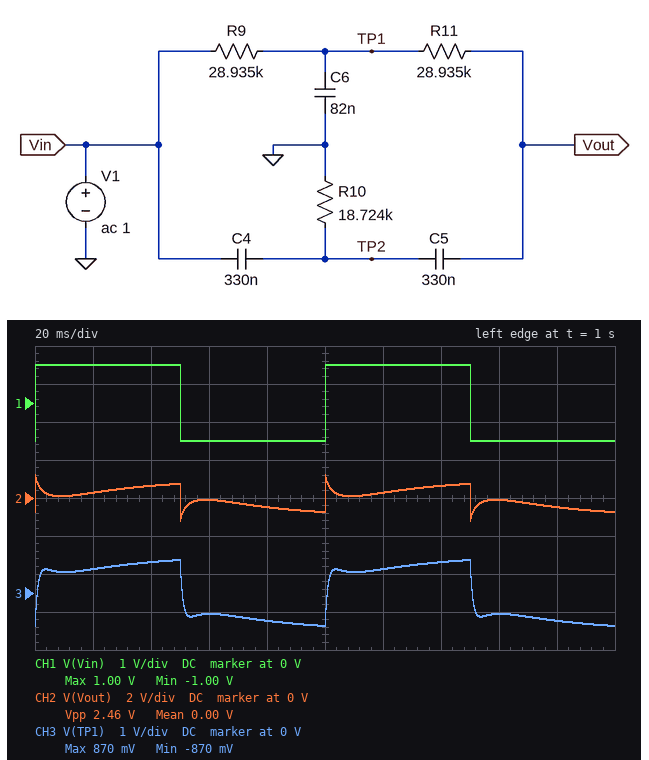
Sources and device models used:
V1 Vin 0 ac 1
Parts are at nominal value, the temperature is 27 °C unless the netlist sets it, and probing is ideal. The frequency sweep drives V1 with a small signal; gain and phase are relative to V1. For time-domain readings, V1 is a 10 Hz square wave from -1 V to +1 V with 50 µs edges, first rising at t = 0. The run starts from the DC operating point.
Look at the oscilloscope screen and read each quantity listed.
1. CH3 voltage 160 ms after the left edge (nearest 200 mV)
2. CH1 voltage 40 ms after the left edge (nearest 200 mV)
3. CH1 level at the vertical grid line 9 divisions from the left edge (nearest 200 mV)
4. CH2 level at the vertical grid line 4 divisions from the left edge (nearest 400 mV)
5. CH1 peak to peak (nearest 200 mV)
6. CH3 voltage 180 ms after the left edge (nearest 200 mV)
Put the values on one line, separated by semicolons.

-600 mV; 1.0 V; -1.0 V; -400 mV; 2.0 V; -800 mV
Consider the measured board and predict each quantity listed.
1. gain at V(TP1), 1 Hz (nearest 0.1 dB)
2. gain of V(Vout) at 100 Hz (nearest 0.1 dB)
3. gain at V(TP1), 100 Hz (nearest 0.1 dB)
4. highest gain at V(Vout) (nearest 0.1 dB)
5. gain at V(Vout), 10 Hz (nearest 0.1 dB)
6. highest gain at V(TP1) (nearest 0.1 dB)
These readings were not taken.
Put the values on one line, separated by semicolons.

-0.1 dB; -2.1 dB; -3.0 dB; 0 dB; -7.3 dB; 0 dB
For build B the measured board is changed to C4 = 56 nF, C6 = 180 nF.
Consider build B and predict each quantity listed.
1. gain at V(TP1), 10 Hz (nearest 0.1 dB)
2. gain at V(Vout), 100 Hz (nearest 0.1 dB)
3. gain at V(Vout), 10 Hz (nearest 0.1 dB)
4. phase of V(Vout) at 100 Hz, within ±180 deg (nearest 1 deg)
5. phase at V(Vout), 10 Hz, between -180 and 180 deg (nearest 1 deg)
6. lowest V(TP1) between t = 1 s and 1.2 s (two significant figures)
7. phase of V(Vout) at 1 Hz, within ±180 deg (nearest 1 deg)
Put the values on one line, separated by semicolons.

-3.3 dB; -11.7 dB; -6.1 dB; 60 deg; -48 deg; -860 mV; -9 deg
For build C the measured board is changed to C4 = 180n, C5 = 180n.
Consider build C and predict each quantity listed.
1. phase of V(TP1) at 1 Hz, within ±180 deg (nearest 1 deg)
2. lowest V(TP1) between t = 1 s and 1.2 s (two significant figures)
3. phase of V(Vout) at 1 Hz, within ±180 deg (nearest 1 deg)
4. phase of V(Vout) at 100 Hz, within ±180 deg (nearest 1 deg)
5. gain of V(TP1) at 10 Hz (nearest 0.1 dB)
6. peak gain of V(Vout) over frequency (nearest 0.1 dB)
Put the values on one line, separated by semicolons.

-3 deg; -960 mV; -5 deg; 30 deg; -1.9 dB; 0 dB
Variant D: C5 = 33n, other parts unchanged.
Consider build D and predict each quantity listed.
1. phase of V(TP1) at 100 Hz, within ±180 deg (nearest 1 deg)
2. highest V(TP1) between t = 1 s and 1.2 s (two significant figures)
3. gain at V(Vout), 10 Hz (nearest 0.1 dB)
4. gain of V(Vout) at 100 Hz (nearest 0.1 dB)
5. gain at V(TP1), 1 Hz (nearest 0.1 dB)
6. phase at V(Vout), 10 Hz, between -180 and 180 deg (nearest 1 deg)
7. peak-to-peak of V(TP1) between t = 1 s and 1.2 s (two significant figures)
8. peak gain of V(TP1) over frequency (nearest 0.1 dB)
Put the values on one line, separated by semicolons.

-35 deg; 1.0 V; -0.6 dB; -9.7 dB; 0 dB; -14 deg; 2.0 V; 0 dB
